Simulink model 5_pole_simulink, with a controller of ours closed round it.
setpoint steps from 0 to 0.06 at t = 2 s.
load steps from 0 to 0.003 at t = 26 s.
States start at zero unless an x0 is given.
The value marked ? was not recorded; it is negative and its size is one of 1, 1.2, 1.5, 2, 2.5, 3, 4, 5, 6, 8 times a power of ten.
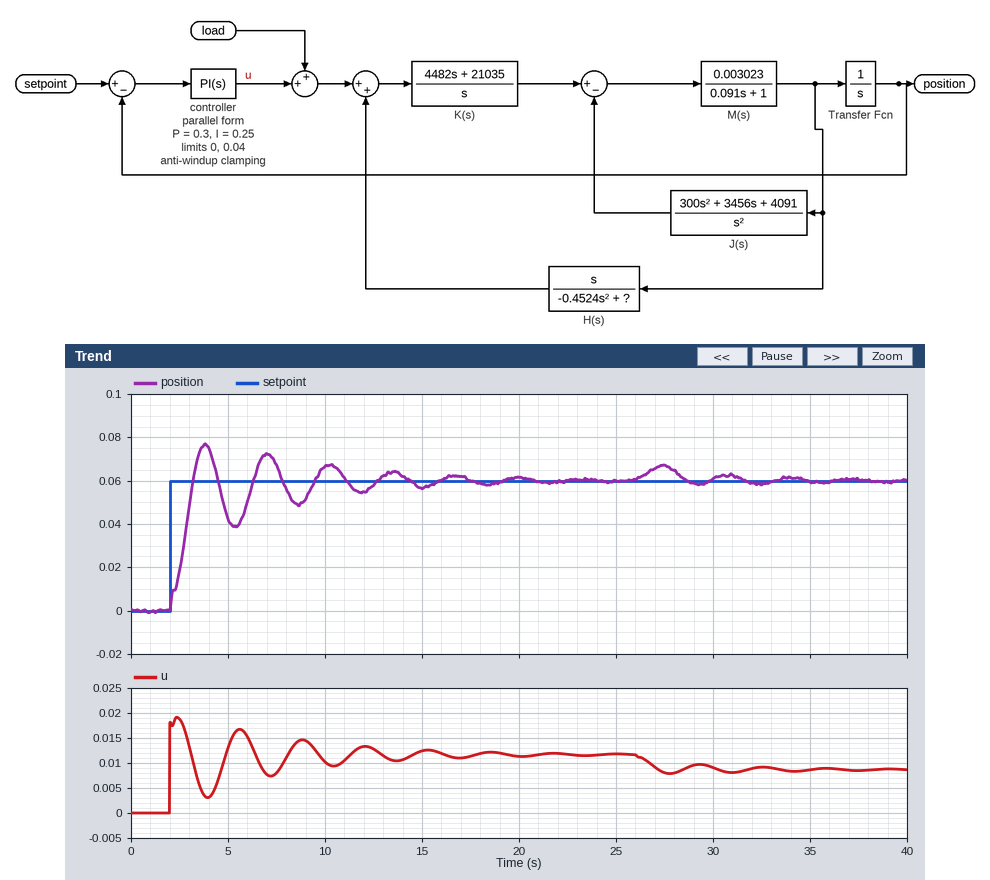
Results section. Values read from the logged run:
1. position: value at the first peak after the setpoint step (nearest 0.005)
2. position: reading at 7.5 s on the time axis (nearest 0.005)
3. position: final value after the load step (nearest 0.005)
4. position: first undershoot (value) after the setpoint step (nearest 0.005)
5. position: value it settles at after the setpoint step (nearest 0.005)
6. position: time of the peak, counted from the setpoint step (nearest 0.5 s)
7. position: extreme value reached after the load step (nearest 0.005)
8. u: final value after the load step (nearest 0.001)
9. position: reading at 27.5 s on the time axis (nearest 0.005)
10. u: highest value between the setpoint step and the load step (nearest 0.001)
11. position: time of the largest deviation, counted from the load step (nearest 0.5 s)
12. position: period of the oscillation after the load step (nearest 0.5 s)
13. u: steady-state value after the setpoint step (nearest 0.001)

0.075
0.065
0.060
0.040
0.060
2.0 s
0.065
0.009
0.065
0.019
1.5 s
3.5 s
0.012
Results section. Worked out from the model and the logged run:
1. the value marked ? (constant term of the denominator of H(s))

-10
